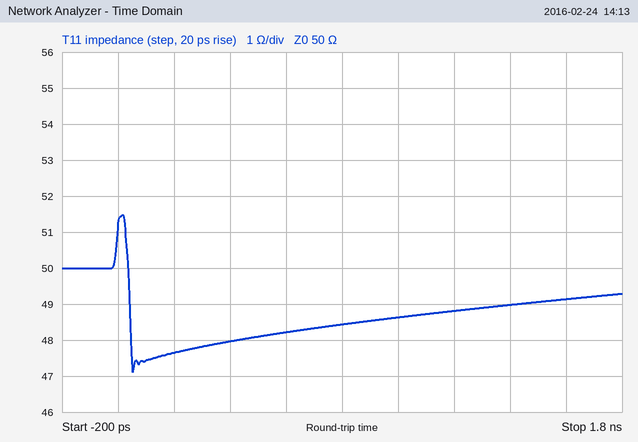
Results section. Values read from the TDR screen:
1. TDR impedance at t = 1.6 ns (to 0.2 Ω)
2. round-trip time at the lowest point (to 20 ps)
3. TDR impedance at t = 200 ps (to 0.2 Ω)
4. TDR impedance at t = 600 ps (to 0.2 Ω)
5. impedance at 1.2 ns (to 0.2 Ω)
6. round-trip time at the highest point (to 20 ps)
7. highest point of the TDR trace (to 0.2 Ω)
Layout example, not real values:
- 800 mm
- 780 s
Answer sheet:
- 49.2 Ω
- 60 ps
- 47.6 Ω
- 48.2 Ω
- 48.8 Ω
- 20 ps
- 51.4 Ω
